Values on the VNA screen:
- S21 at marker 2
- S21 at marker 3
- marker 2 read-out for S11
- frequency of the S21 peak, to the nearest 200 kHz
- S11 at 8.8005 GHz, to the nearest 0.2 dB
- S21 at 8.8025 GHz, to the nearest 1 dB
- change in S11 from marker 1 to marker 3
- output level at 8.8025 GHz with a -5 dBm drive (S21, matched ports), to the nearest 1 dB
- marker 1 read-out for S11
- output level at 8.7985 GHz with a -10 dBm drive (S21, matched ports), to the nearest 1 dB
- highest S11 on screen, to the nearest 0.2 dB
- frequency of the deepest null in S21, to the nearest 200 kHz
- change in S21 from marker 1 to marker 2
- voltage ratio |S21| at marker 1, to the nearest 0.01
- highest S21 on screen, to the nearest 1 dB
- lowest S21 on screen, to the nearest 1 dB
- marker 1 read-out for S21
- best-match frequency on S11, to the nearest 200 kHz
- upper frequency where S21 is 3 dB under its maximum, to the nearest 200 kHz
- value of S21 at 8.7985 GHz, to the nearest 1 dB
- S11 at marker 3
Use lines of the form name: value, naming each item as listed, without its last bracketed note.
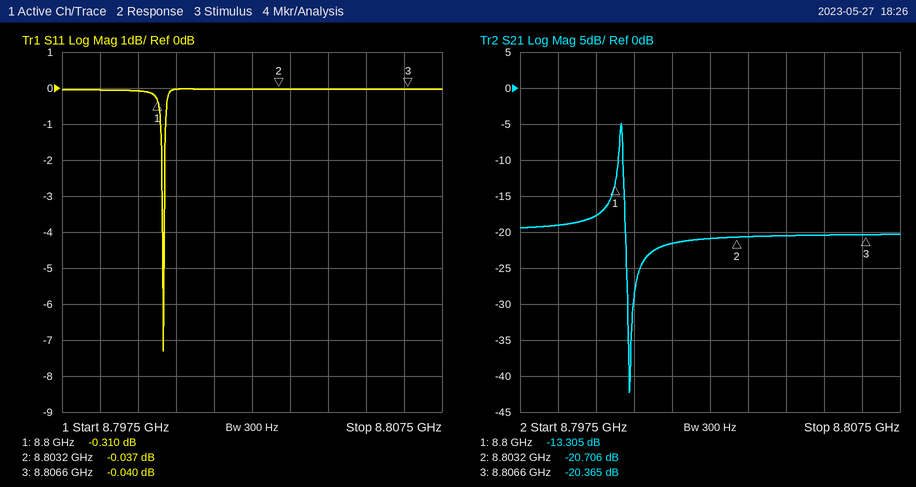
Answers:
S21 at marker 2: -20.706 dB
S21 at marker 3: -20.365 dB
marker 2 read-out for S11: -0.037 dB
frequency of the S21 peak, to the nearest 200 kHz: 8.8002 GHz
S11 at 8.8005 GHz, to the nearest 0.2 dB: 0.0 dB
S21 at 8.8025 GHz, to the nearest 1 dB: -21 dB
change in S11 from marker 1 to marker 3: 0.270 dB
output level at 8.8025 GHz with a -5 dBm drive (S21, matched ports), to the nearest 1 dB: -26 dBm
marker 1 read-out for S11: -0.310 dB
output level at 8.7985 GHz with a -10 dBm drive (S21, matched ports), to the nearest 1 dB: -29 dBm
highest S11 on screen, to the nearest 0.2 dB: 0.0 dB
frequency of the deepest null in S21, to the nearest 200 kHz: 8.8004 GHz
change in S21 from marker 1 to marker 2: -7.401 dB
voltage ratio |S21| at marker 1, to the nearest 0.01: 0.22
highest S21 on screen, to the nearest 1 dB: -5 dB
lowest S21 on screen, to the nearest 1 dB: -42 dB
marker 1 read-out for S21: -13.305 dB
best-match frequency on S11, to the nearest 200 kHz: 8.8002 GHz
upper frequency where S21 is 3 dB under its maximum, to the nearest 200 kHz: 8.8002 GHz
value of S21 at 8.7985 GHz, to the nearest 1 dB: -19 dB
S11 at marker 3: -0.040 dB
